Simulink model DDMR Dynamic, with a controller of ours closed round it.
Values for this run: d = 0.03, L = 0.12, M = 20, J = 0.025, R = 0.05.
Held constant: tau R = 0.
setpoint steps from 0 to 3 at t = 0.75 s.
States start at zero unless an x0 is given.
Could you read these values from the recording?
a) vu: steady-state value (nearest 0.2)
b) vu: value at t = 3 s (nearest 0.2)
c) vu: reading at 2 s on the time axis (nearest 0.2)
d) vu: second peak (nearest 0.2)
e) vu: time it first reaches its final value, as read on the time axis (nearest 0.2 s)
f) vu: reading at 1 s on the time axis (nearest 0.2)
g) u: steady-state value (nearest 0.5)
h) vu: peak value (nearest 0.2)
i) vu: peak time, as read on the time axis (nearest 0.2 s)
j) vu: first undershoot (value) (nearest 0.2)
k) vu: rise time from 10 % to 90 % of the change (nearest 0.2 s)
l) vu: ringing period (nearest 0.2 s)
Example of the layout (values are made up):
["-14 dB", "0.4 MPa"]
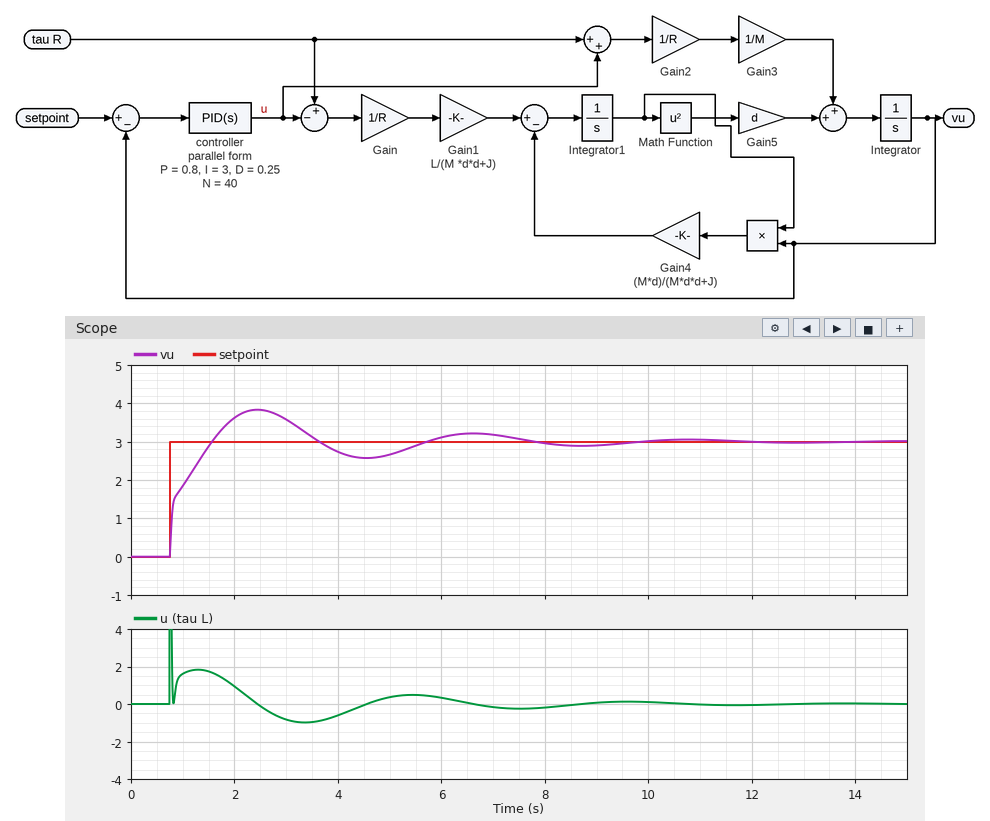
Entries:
["3.0", "3.6", "3.6", "3.2", "1.6 s", "1.8", "0.0", "3.8", "2.4 s", "2.6", "0.6 s", "4.2 s"]
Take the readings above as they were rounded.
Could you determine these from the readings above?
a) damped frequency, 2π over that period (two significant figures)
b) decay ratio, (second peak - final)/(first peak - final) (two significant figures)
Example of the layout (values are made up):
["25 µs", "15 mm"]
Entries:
["1.5 rad/s", "0.25"]
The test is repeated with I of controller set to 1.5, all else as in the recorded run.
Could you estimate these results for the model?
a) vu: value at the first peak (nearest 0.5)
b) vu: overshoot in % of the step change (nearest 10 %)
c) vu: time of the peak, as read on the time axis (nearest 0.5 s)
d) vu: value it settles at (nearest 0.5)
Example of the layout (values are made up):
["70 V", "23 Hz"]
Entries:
["3.5", "20 %", "3.0 s", "3.0"]
